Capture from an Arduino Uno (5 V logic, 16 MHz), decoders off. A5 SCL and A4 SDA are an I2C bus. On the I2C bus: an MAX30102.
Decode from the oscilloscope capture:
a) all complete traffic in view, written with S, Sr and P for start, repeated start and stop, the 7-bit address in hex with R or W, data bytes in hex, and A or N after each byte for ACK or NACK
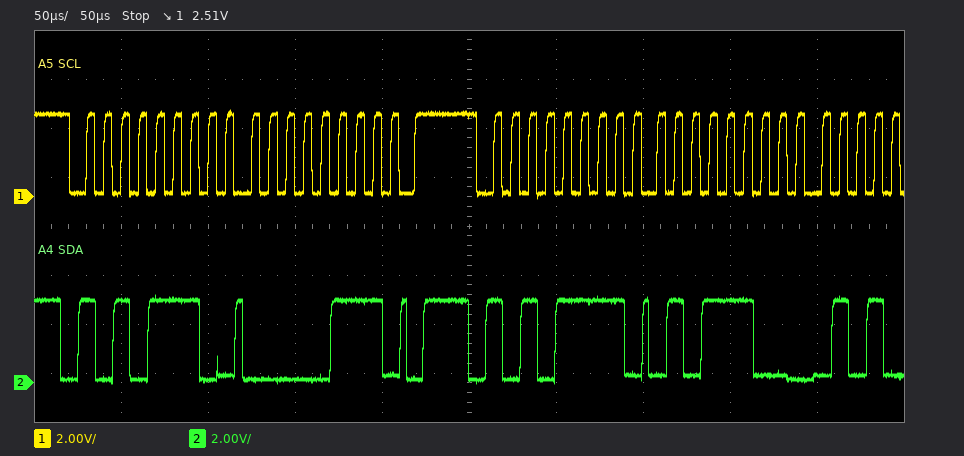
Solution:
S 57W A 07 A P S 57R A 5C A
